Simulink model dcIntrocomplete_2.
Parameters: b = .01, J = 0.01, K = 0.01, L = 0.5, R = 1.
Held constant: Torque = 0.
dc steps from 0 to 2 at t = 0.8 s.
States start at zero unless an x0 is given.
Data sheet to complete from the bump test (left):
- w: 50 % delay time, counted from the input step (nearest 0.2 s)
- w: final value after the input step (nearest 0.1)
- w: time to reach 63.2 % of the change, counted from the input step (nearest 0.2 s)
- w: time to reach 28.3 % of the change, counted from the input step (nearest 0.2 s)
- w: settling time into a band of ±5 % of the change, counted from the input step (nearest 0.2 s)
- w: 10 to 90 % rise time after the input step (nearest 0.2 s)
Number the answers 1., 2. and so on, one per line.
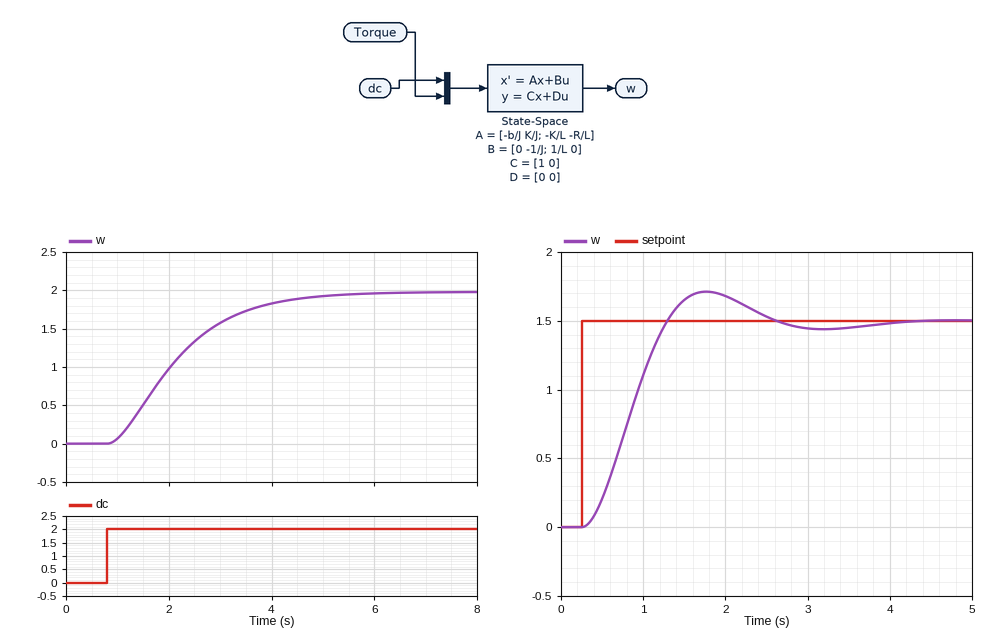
1. 1.2 s
2. 2.0
3. 1.6 s
4. 0.8 s
5. 3.6 s
6. 2.6 s
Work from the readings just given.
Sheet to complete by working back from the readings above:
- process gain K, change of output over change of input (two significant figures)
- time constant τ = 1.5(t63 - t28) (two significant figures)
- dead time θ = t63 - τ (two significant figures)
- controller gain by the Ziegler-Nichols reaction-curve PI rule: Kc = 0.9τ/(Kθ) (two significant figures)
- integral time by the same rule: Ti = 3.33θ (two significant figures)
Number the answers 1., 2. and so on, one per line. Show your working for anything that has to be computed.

1. (2 - 0) / 2 = 1.0
2. 1.5 × (1.6 - 0.8) = 1.2 s
3. 1.6 - 1.2 = 0.40 s
4. 0.9 × 1.2 / (1 × 0.4) = 2.7
5. 3.33 × 0.4 = 1.3 s
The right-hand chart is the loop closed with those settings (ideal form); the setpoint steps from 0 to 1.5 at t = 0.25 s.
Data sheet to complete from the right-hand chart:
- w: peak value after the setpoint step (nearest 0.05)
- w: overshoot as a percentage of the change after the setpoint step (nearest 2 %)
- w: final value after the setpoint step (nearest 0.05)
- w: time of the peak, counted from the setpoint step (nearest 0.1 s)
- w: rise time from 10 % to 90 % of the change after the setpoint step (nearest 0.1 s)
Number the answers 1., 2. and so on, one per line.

1. 1.70
2. 14 %
3. 1.50
4. 1.5 s
5. 0.7 s
